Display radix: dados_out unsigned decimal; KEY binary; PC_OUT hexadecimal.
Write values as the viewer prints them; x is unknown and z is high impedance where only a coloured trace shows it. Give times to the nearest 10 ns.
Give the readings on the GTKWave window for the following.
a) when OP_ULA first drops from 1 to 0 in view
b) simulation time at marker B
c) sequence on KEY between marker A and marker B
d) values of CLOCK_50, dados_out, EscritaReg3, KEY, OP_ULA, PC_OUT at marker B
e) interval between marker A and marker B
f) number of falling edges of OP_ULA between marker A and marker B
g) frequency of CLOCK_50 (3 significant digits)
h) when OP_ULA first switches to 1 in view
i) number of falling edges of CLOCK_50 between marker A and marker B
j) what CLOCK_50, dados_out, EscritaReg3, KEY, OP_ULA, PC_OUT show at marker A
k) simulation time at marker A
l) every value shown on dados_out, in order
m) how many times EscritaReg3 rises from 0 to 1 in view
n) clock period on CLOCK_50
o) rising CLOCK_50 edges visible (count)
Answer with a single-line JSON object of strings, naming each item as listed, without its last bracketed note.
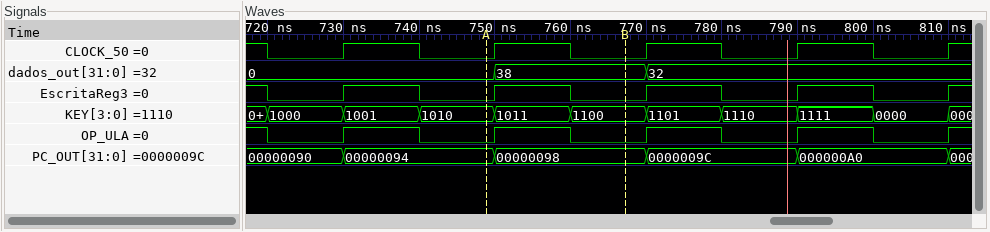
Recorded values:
{"when OP_ULA first drops from 1 to 0 in view": "720 ns", "simulation time at marker B": "770 ns", "sequence on KEY between marker A and marker B": "1010, 1011, 1100", "values of CLOCK_50, dados_out, EscritaReg3, KEY, OP_ULA, PC_OUT at marker B": "CLOCK_50=0, dados_out=38, EscritaReg3=0, KEY=1100, OP_ULA=0, PC_OUT=00000098", "interval between marker A and marker B": "20 ns", "number of falling edges of OP_ULA between marker A and marker B": "1", "frequency of CLOCK_50": "50.0 MHz", "when OP_ULA first switches to 1 in view": "730 ns", "number of falling edges of CLOCK_50 between marker A and marker B": "1", "what CLOCK_50, dados_out, EscritaReg3, KEY, OP_ULA, PC_OUT show at marker A": "CLOCK_50=0, dados_out=0, EscritaReg3=0, KEY=1010, OP_ULA=0, PC_OUT=00000094", "simulation time at marker A": "750 ns", "every value shown on dados_out, in order": "0, 38, 32", "how many times EscritaReg3 rises from 0 to 1 in view": "5", "clock period on CLOCK_50": "20 ns", "rising CLOCK_50 edges visible": "5"}
